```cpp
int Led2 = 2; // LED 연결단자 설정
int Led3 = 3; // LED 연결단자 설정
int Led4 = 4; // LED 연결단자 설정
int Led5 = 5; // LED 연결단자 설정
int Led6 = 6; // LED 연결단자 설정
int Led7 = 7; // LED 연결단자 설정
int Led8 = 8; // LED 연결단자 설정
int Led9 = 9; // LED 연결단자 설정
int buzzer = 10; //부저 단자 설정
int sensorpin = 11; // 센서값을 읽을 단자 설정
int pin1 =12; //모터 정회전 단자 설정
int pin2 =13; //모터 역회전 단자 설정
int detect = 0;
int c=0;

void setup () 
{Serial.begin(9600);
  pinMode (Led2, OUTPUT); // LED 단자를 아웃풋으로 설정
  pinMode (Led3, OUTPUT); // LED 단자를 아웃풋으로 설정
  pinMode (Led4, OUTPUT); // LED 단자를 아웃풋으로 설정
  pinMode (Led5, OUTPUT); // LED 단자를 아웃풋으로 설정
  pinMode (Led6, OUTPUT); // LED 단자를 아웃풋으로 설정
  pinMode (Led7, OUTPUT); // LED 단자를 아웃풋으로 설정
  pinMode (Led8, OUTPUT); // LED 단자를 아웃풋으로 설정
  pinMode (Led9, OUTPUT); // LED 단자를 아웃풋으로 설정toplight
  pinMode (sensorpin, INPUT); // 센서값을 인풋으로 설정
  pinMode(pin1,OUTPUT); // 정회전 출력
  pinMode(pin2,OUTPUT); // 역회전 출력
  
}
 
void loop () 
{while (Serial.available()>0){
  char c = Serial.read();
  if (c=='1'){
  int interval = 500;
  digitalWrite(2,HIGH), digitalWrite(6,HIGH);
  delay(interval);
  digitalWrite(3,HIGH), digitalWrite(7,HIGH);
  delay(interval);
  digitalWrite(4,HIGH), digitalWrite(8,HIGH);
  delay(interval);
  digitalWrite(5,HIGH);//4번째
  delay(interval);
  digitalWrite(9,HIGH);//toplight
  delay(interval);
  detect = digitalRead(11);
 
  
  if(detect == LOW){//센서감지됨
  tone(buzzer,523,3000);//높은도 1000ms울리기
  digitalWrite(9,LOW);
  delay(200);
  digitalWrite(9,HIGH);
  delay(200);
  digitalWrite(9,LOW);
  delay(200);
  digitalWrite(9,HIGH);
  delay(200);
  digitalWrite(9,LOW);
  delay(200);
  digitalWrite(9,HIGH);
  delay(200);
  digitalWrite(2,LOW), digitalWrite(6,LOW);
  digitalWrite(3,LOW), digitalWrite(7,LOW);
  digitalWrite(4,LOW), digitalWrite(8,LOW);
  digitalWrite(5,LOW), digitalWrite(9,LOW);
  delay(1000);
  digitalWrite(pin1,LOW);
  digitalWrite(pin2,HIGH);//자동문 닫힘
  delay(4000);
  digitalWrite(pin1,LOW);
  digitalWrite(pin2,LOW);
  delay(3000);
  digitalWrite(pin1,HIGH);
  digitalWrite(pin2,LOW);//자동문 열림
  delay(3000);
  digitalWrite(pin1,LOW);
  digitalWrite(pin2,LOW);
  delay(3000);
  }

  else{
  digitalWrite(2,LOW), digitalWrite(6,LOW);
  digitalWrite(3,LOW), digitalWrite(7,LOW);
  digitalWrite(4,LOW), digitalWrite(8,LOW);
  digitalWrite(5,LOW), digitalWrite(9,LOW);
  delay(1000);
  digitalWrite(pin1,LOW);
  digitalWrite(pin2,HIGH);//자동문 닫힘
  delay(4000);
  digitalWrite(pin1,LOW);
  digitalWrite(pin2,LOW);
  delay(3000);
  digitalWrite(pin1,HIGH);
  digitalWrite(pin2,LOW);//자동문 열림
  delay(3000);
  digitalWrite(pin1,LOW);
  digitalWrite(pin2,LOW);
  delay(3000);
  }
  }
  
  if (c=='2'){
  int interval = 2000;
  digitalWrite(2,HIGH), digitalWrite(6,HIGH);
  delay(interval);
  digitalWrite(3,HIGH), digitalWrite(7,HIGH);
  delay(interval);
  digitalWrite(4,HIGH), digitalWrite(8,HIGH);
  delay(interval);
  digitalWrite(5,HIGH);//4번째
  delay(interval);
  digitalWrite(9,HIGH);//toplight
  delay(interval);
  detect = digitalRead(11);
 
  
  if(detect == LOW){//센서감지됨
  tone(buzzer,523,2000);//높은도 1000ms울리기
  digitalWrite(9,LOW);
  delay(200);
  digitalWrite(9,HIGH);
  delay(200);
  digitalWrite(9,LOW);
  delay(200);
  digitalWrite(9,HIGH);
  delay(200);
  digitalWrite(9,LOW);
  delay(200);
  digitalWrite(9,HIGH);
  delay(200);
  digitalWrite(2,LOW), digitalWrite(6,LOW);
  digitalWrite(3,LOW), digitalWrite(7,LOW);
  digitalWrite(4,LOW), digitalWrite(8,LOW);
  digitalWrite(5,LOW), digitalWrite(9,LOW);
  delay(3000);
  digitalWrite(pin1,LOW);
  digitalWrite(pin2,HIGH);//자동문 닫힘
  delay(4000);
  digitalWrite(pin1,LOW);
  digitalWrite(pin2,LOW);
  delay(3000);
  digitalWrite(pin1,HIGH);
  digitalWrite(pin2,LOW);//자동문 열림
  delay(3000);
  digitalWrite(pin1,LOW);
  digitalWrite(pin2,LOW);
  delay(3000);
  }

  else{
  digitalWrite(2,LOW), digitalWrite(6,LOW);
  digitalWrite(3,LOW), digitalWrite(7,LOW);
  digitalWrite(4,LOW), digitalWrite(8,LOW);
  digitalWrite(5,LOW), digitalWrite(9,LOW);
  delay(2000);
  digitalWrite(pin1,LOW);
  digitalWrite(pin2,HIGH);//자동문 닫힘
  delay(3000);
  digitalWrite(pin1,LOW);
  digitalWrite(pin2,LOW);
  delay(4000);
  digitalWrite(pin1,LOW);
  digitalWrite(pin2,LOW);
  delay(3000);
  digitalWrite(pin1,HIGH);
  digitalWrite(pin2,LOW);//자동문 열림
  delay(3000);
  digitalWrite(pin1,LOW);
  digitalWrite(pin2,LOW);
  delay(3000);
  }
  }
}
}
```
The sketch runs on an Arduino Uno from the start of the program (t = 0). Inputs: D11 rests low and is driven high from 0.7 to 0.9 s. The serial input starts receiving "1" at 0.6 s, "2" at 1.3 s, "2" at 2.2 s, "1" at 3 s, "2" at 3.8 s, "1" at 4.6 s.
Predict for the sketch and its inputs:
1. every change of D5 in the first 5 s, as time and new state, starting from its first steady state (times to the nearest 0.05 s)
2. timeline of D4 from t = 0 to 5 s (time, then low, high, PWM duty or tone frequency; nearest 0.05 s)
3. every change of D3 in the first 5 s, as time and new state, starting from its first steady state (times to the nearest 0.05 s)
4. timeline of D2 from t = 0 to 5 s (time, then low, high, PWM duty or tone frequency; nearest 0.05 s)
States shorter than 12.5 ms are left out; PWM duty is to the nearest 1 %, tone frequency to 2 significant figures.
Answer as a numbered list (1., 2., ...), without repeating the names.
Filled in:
1. 0 s low; 2.1 s high; 4.3 s low
2. 0 s low; 1.6 s high; 4.3 s low
3. 0 s low; 1.1 s high; 4.3 s low
4. 0 s low; 0.6 s high; 4.3 s low
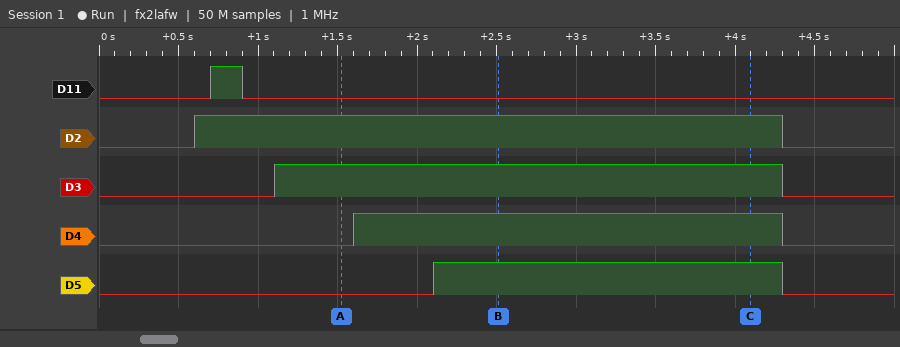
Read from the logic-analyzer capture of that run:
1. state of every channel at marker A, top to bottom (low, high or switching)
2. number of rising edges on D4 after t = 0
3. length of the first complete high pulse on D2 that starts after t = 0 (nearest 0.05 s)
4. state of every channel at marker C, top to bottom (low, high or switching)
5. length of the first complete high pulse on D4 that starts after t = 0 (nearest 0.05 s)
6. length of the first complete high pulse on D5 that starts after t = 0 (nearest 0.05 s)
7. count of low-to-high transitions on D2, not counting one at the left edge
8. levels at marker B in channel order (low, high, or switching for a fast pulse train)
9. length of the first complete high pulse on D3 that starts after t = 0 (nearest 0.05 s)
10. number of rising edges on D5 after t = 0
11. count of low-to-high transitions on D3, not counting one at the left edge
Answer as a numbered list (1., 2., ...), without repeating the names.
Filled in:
1. D11 low, D2 high, D3 high, D4 low, D5 low
2. 1
3. 3.70 s
4. D11 low, D2 high, D3 high, D4 high, D5 high
5. 2.70 s
6. 2.20 s
7. 1
8. D11 low, D2 high, D3 high, D4 high, D5 high
9. 3.20 s
10. 1
11. 1
